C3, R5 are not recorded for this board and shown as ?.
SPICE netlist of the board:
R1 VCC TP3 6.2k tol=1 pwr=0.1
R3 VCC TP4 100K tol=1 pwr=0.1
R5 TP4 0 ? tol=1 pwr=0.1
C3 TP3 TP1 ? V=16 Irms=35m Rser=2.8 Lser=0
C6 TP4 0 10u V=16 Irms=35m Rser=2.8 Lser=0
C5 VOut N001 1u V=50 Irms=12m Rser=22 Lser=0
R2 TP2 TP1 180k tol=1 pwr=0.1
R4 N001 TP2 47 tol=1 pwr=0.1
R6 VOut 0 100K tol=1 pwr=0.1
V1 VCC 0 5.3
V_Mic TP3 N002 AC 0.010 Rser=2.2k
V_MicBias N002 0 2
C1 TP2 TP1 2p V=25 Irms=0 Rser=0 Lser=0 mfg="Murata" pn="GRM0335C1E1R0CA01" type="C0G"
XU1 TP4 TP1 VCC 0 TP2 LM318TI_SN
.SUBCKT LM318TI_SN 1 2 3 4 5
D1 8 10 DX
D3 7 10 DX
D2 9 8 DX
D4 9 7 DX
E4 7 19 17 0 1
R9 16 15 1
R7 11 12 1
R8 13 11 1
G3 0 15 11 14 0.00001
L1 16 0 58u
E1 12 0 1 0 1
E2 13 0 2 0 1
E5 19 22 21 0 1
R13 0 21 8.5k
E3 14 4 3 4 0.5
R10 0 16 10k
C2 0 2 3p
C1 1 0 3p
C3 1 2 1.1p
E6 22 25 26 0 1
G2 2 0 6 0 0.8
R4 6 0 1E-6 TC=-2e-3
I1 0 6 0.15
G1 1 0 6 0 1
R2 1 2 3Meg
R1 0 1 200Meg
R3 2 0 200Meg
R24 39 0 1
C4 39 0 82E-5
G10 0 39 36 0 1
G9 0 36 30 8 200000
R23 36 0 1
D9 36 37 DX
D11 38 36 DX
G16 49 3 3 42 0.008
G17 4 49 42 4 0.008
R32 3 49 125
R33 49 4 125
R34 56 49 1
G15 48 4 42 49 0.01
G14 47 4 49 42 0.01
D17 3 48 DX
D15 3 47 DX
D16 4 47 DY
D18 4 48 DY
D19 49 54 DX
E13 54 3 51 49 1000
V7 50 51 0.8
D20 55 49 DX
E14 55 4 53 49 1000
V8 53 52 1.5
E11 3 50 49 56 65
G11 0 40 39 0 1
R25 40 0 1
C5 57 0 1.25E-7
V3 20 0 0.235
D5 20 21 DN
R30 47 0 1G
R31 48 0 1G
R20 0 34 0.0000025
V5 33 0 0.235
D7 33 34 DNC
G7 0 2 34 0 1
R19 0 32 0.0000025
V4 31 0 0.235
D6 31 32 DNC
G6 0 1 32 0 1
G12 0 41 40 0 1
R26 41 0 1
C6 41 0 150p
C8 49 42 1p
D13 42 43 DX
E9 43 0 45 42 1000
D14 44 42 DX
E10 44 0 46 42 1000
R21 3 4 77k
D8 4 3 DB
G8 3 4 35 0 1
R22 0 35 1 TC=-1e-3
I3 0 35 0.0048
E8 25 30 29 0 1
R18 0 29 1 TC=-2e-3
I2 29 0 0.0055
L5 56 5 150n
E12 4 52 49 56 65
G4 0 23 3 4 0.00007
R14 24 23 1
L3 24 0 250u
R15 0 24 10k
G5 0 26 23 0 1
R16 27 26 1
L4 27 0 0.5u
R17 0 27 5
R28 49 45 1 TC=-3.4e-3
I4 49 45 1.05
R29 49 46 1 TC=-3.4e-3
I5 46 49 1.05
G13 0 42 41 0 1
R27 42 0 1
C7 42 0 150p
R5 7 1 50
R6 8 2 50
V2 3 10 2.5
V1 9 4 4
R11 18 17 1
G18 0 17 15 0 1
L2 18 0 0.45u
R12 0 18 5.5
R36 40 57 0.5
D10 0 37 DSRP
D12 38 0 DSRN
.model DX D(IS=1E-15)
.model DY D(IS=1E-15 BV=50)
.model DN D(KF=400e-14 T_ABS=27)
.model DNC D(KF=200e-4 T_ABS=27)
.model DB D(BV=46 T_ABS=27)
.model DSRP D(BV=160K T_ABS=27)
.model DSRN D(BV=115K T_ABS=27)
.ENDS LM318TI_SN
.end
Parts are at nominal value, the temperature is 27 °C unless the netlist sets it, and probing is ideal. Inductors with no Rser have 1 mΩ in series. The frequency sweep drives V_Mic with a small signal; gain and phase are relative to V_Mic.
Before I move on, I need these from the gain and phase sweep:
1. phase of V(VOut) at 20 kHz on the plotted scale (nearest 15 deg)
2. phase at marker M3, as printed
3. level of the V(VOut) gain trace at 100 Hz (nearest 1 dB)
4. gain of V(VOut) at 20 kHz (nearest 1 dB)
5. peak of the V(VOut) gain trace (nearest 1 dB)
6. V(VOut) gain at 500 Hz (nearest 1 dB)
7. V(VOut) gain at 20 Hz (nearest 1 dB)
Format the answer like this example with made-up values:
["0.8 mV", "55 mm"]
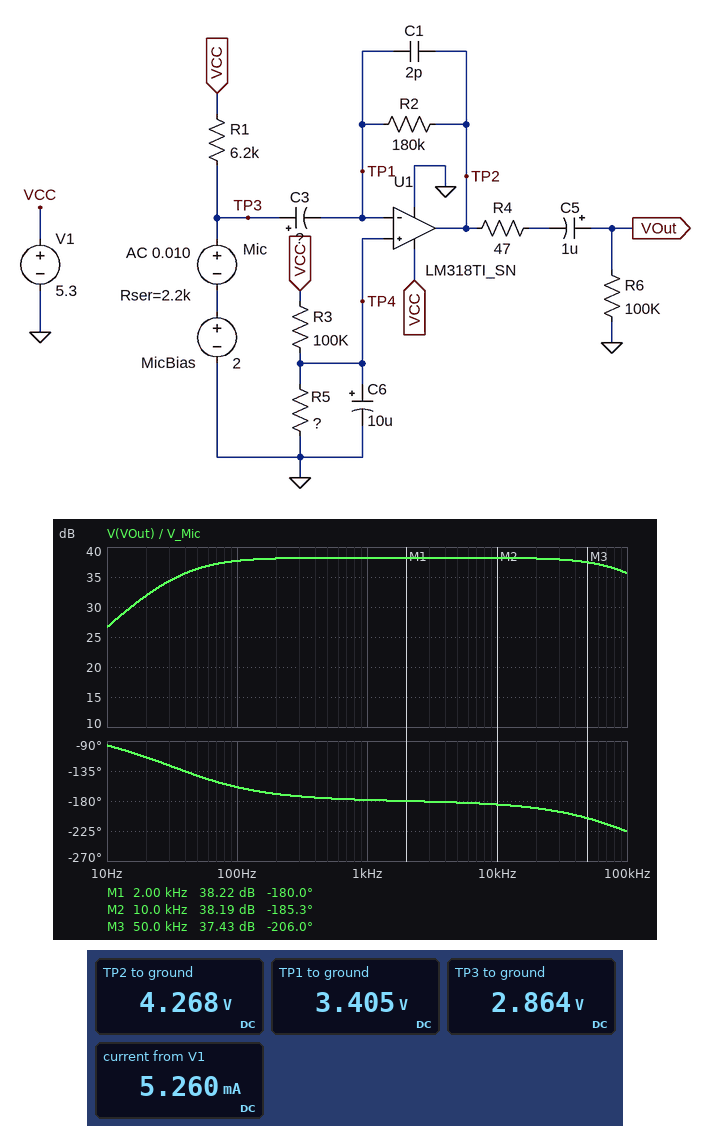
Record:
["-195 deg", "-206.0 deg", "38 dB", "38 dB", "38 dB", "38 dB", "32 dB"]
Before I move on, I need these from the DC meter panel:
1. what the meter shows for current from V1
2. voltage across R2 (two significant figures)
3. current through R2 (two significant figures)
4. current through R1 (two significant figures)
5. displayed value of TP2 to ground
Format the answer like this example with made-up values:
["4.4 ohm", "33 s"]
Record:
["5.260 mA", "860 mV", "4.8 µA", "390 µA", "4.268 V"]
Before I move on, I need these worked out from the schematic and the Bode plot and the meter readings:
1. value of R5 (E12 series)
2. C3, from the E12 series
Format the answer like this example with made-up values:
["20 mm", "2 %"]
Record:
["180 kΩ", "2.7 µF"]
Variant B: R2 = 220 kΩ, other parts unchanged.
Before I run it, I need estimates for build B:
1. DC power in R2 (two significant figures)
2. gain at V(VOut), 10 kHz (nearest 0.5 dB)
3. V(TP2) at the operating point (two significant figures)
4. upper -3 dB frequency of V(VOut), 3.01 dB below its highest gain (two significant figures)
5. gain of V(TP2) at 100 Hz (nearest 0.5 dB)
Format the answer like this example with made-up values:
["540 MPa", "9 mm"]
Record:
["5.1 µW", "40.0 dB", "4.5 V", "90 kHz", "39.5 dB"]
